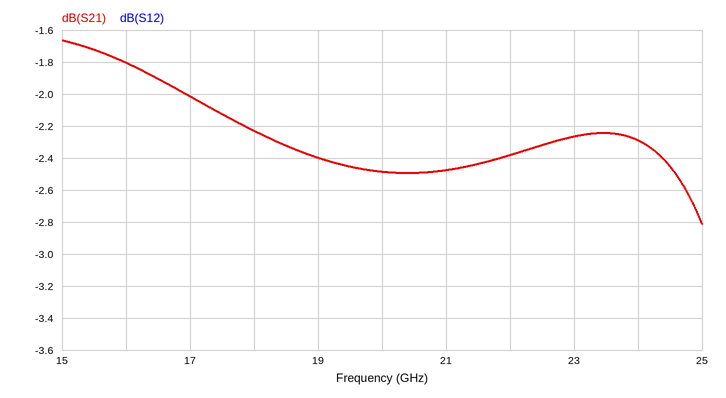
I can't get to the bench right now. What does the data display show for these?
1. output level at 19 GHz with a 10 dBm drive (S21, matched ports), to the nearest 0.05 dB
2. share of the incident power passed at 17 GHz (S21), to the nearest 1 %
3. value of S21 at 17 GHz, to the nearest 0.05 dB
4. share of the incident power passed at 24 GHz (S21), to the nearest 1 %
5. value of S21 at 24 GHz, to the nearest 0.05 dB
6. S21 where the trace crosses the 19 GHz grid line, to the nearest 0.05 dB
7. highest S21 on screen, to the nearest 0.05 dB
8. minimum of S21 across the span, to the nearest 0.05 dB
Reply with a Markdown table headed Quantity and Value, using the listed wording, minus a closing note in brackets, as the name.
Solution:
| Quantity | Value |
|---|---|
| output level at 19 GHz with a 10 dBm drive (S21, matched ports), to the nearest 0.05 dB | 7.60 dBm |
| share of the incident power passed at 17 GHz (S21), to the nearest 1 % | 63 % |
| value of S21 at 17 GHz, to the nearest 0.05 dB | -2.00 dB |
| share of the incident power passed at 24 GHz (S21), to the nearest 1 % | 59 % |
| value of S21 at 24 GHz, to the nearest 0.05 dB | -2.30 dB |
| S21 where the trace crosses the 19 GHz grid line, to the nearest 0.05 dB | -2.40 dB |
| highest S21 on screen, to the nearest 0.05 dB | -1.65 dB |
| minimum of S21 across the span, to the nearest 0.05 dB | -2.80 dB |
